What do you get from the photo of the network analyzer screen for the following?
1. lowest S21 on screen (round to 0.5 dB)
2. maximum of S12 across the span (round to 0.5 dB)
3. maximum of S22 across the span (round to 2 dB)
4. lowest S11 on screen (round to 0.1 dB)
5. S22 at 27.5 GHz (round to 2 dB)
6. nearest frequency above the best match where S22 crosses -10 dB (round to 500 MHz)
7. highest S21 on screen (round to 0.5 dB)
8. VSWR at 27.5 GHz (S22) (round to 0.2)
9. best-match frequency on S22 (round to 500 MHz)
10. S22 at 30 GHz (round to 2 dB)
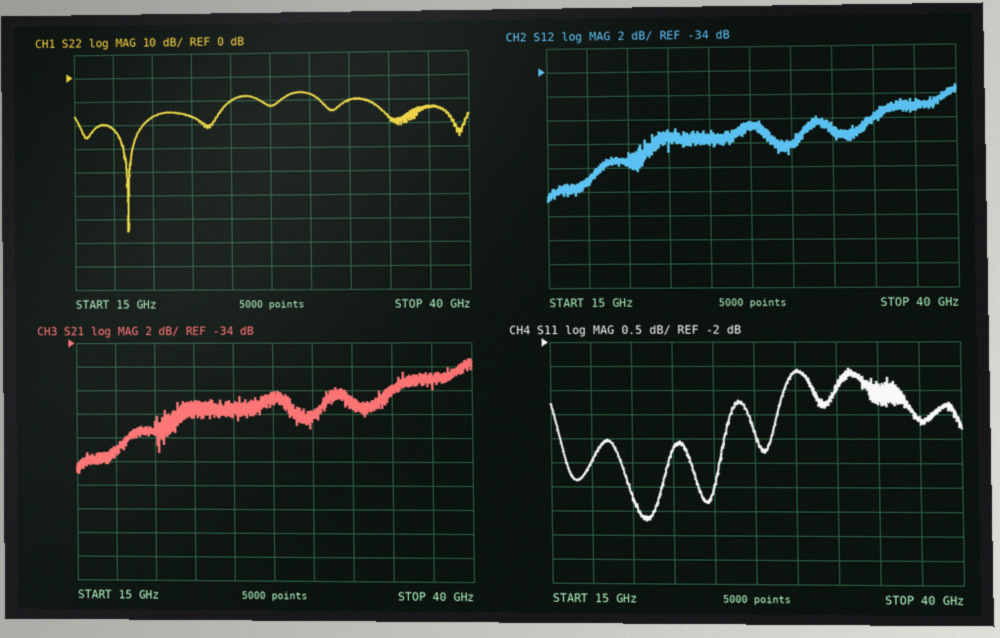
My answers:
-45.0 dB
-35.5 dB
-6 dB
-5.7 dB
-12 dB
25.0 GHz
-35.5 dB
1.6
18.5 GHz
-8 dB
